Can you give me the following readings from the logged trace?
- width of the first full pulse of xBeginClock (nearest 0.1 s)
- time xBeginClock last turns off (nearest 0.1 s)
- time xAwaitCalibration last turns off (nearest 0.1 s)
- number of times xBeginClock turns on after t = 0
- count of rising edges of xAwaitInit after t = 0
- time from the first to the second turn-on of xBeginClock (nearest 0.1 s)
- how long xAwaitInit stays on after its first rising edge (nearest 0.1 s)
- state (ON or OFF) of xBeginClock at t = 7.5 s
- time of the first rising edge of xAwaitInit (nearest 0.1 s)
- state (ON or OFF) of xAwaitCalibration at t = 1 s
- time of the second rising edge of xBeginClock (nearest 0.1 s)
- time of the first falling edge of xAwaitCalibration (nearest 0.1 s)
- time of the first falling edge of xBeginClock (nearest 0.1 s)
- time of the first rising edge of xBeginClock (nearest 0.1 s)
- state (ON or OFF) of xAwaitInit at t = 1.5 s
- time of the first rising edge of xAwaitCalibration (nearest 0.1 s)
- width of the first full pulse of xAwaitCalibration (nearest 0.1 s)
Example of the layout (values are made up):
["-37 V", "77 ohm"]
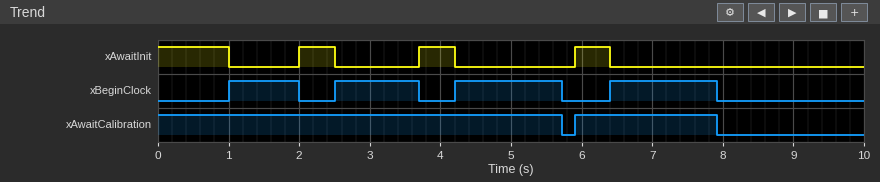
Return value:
["1.0 s", "7.9 s", "7.9 s", "4", "3", "1.5 s", "0.5 s", "ON", "2.0 s", "ON", "2.5 s", "5.7 s", "2.0 s", "1.0 s", "OFF", "5.9 s", "2.0 s"]
